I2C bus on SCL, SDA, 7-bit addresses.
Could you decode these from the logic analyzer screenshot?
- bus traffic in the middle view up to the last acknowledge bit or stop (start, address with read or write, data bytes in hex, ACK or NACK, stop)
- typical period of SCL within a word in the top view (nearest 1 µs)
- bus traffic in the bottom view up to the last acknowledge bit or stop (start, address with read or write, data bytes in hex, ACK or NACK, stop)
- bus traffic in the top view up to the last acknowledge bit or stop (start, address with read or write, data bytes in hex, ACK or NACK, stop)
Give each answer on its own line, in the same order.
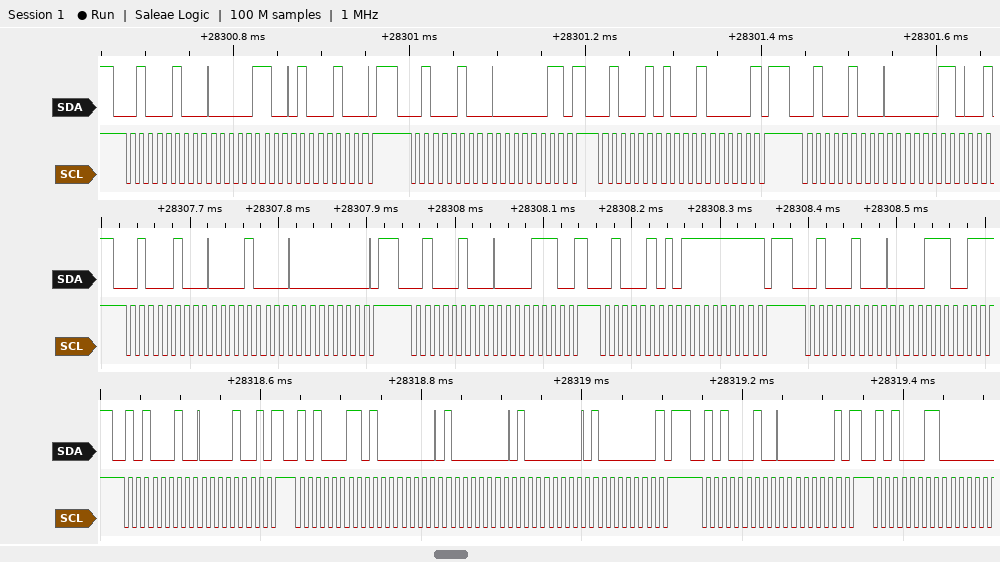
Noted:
start, address 22 write ACK, 08 ACK, 00 ACK, stop, start, address 22 write ACK, 0E ACK, repeated start, address 22 read ACK, FF NACK, stop, start, address 22 write ACK, 0E ACK
10 µs
start, address 51 write ACK, 09 ACK, repeated start, address 51 read ACK, 80 ACK, 80 ACK, 80 ACK, 80 NACK, stop, start, address 51 write ACK, 01 ACK, repeated start, address 51 read ACK
start, address 22 write ACK, 06 ACK, 44 ACK, stop, start, address 22 write ACK, 03 ACK, repeated start, address 22 read ACK, 20 NACK, stop, start, address 22 write ACK, 03 ACK
